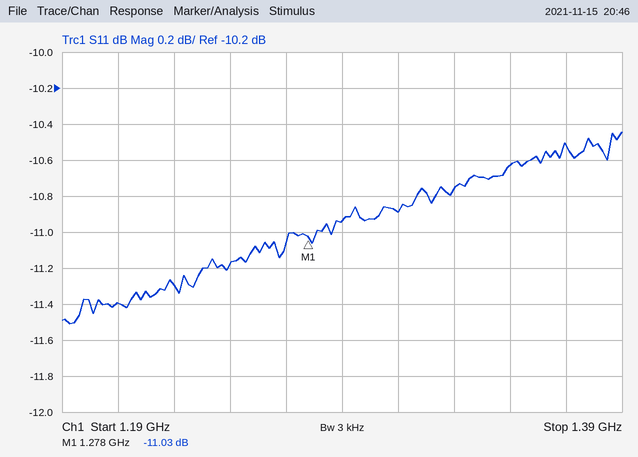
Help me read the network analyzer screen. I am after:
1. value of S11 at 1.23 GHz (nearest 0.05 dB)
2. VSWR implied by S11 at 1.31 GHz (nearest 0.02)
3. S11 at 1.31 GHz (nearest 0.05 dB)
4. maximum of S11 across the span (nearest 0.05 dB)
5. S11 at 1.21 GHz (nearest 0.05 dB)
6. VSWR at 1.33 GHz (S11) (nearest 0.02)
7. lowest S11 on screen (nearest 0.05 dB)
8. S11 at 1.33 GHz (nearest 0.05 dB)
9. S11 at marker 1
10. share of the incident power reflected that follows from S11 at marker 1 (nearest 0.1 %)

-11.30 dB
1.80
-10.90 dB
-10.45 dB
-11.40 dB
1.82
-11.50 dB
-10.75 dB
-11.03 dB
7.9 %
